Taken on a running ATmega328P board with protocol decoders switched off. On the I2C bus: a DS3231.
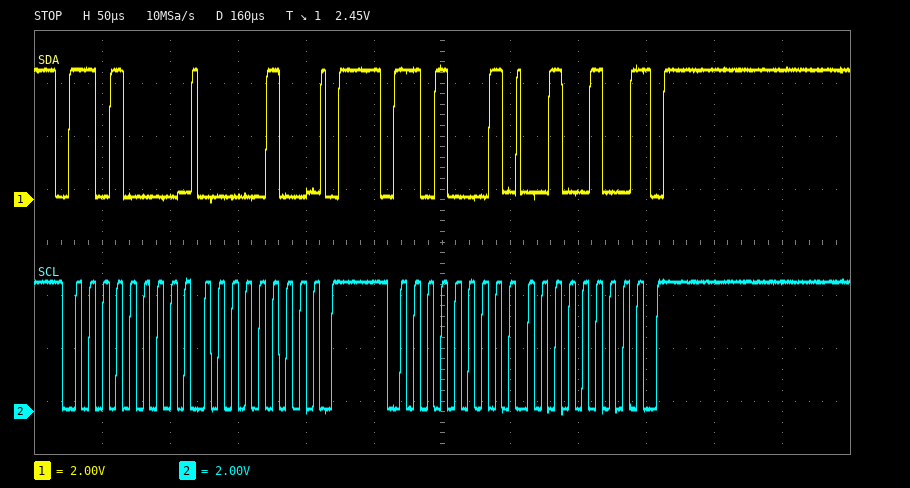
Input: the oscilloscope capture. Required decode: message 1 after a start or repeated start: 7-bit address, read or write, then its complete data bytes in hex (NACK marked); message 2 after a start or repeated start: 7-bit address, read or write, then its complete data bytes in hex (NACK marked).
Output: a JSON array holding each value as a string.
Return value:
["0x68 write: 04", "0x68 read: 24 NACK"]
